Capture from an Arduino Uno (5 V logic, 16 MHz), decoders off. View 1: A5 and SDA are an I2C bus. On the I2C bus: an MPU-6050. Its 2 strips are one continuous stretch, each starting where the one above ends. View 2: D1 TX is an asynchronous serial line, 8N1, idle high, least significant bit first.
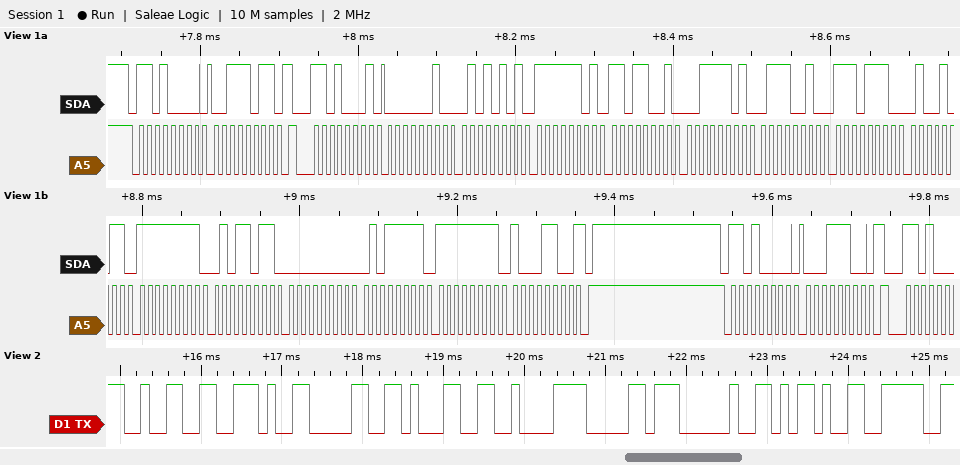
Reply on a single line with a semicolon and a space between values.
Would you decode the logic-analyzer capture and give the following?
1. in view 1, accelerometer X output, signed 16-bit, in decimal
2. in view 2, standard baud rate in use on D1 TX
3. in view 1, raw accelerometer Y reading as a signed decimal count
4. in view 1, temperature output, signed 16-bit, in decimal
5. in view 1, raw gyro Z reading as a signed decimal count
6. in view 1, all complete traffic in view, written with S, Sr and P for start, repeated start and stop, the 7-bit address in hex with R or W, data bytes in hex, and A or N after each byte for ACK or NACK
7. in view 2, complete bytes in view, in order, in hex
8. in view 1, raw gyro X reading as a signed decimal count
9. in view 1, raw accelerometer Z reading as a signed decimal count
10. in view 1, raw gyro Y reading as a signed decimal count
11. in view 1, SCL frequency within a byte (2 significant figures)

597; 9600 baud; -551; -4533; -116; S 68W A 3B A Sr 68R A 02 A 55 A FD A D9 A 3D A 72 A EE A 4B A FF A 5B A 00 A 5F A FF A 8C N P S 68W A 1C A; 32 2E 30 31 C2 B0 20 2D 3E; -165; 15730; 95; 100 kHz
